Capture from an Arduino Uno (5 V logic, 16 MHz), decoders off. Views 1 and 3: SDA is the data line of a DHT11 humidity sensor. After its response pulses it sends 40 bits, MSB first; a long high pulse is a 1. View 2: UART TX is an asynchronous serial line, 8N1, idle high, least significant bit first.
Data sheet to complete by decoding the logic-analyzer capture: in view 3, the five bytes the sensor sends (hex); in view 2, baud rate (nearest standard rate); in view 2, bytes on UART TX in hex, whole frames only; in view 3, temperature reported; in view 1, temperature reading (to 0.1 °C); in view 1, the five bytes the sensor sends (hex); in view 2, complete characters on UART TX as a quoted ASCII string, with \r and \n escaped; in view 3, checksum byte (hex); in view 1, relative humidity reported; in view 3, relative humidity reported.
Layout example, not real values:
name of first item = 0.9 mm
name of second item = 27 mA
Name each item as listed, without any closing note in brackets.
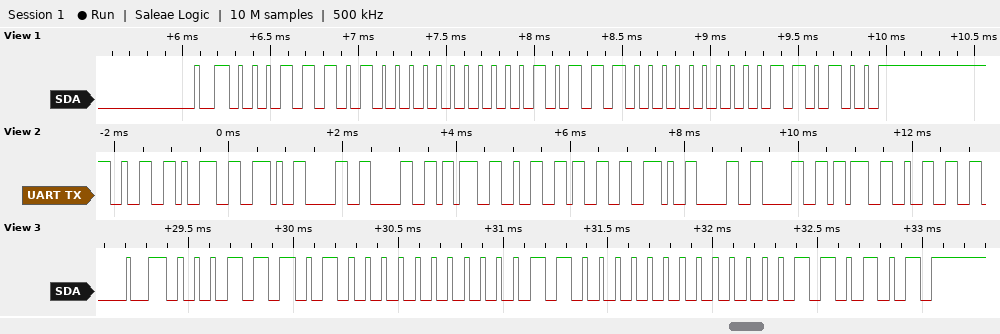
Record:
in view 3, the five bytes the sensor sends = 1D 00 18 00 35
in view 2, baud rate = 9600 baud
in view 2, bytes on UART TX in hex, whole frames only = 32 39 2E 30 30 3B 32 33 2E 30 30 3B 32
in view 3, temperature reported = 24.0 °C
in view 1, temperature reading = 23.0 °C
in view 1, the five bytes the sensor sends = 1D 00 17 00 34
in view 2, complete characters on UART TX as a quoted ASCII string, with \r and \n escaped = "29.00;23.00;2"
in view 3, checksum byte = 0x35
in view 1, relative humidity reported = 29 %
in view 3, relative humidity reported = 29 %
